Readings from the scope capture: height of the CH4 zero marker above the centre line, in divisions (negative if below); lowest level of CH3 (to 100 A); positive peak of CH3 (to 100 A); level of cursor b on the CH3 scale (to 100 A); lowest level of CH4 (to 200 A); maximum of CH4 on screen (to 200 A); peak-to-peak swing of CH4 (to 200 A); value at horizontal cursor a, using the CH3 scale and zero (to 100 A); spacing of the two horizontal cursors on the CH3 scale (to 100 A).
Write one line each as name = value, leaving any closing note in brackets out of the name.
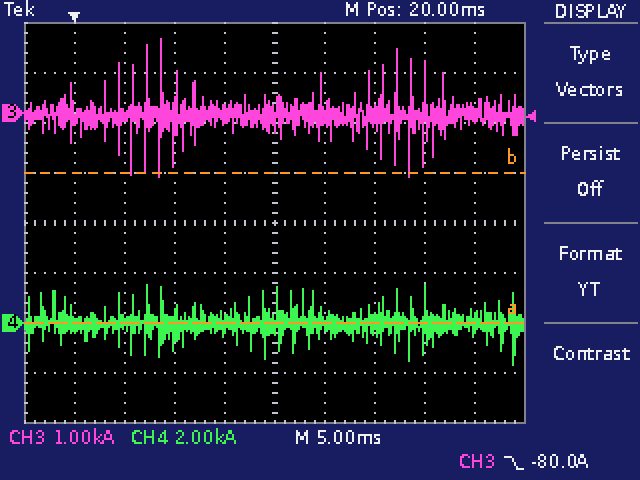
height of the CH4 zero marker above the centre line, in divisions = -2.0 div
lowest level of CH3 = -1.3 kA
positive peak of CH3 = 1.5 kA
level of cursor b on the CH3 scale = -1.2 kA
lowest level of CH4 = -1.6 kA
maximum of CH4 on screen = 1.6 kA
peak-to-peak swing of CH4 = 3.2 kA
value at horizontal cursor a, using the CH3 scale and zero = -4.2 kA
spacing of the two horizontal cursors on the CH3 scale = 3.0 kA
